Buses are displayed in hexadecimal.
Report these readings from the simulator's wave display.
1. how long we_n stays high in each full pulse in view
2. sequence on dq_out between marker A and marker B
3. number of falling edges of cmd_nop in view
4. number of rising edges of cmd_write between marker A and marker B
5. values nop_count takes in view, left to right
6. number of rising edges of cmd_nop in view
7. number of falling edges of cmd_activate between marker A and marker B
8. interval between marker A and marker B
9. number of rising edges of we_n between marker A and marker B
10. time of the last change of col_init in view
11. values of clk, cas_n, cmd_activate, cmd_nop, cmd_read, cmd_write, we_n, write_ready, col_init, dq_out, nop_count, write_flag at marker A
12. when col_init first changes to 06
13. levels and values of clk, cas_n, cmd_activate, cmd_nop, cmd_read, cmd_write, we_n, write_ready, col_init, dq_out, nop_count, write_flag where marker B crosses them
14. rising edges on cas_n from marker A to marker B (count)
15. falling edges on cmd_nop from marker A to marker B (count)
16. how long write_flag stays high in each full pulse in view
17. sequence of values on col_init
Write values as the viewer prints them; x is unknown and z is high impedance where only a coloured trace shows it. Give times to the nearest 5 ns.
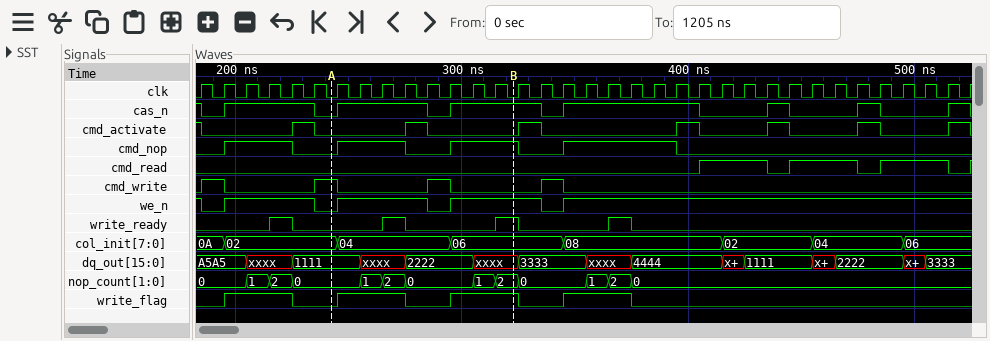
40 ns, 40 ns, 40 ns
1111, xxxx, 2222, xxxx
4
1
0, 1, 2, 0, 1, 2, 0, 1, 2, 0, 1, 2, 0
4
1
80 ns
2
495 ns
clk=0, cas_n=0, cmd_activate=0, cmd_nop=0, cmd_read=0, cmd_write=1, we_n=0, write_ready=0, col_init=02, dq_out=1111, nop_count=0, write_flag=0
295 ns
clk=0, cas_n=1, cmd_activate=0, cmd_nop=1, cmd_read=0, cmd_write=0, we_n=1, write_ready=1, col_init=06, dq_out=xxxx, nop_count=2, write_flag=1
2
1
30 ns, 30 ns, 30 ns, 30 ns
0A, 02, 04, 06, 08, 02, 04, 06
